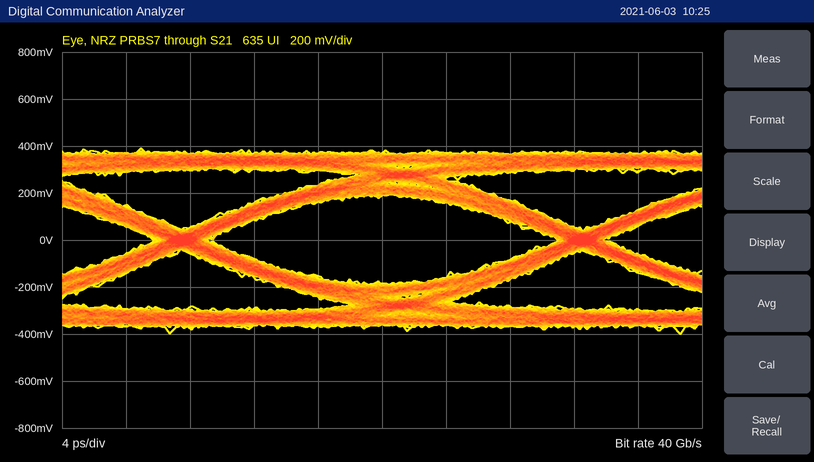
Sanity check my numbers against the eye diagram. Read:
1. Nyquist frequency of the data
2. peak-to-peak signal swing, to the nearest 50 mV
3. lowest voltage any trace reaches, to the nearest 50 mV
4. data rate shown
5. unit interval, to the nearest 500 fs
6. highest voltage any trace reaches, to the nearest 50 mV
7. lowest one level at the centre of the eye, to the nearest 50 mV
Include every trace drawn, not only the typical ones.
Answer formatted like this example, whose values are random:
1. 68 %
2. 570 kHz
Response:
1. 20 GHz
2. 800 mV
3. -400 mV
4. 40 Gb/s
5. 25.0 ps
6. 400 mV
7. 200 mV
